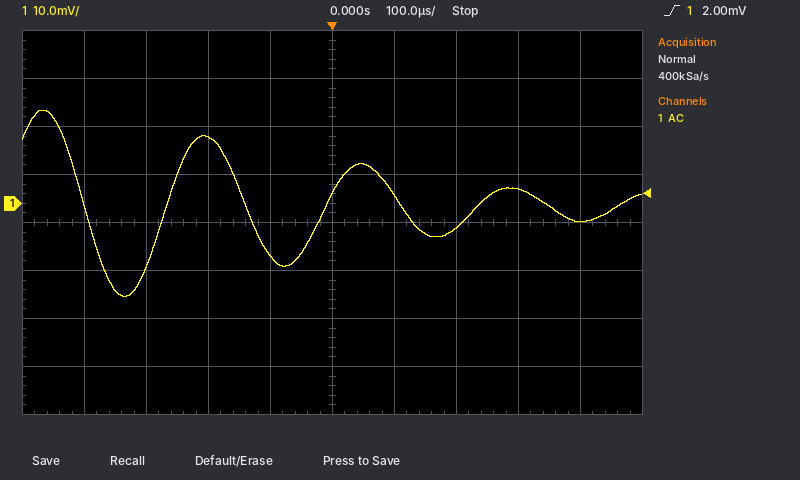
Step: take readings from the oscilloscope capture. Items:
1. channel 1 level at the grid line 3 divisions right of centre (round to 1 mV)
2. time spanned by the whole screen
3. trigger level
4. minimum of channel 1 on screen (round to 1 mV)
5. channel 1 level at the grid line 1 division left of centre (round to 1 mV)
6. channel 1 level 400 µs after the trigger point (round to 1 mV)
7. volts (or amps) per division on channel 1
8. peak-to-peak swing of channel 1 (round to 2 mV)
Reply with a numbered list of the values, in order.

1. 3 mV
2. 1 ms
3. 2.00 mV
4. -19 mV
5. -11 mV
6. -4 mV
7. 10 mV
8. 38 mV
